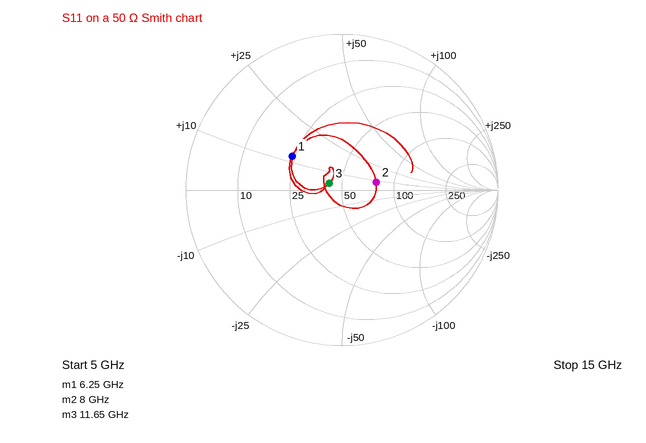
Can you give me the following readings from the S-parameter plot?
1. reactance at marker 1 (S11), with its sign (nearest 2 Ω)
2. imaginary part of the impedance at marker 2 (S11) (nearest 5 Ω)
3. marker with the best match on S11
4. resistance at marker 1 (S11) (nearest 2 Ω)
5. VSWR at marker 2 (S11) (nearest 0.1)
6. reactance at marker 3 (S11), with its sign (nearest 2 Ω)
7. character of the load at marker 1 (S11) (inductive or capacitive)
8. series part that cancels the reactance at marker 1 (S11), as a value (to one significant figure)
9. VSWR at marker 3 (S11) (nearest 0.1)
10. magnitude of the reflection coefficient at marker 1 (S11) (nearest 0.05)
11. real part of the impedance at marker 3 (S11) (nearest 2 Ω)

+12 Ω
+10 Ω
marker 3
24 Ω
1.6
+4 Ω
inductive
2 pF
1.2
0.40
42 Ω
